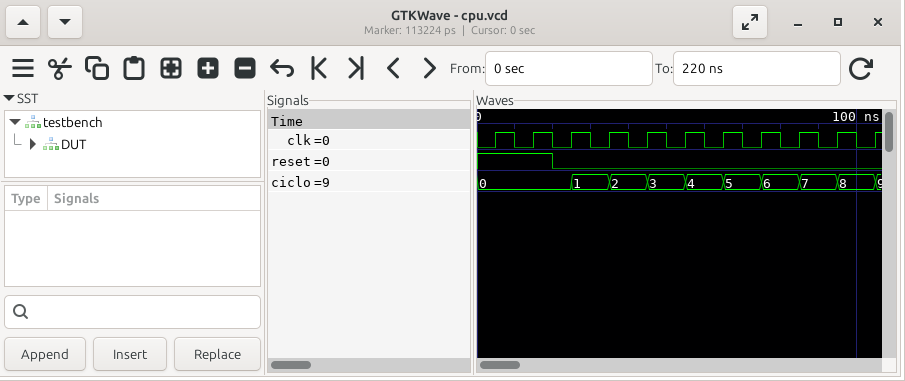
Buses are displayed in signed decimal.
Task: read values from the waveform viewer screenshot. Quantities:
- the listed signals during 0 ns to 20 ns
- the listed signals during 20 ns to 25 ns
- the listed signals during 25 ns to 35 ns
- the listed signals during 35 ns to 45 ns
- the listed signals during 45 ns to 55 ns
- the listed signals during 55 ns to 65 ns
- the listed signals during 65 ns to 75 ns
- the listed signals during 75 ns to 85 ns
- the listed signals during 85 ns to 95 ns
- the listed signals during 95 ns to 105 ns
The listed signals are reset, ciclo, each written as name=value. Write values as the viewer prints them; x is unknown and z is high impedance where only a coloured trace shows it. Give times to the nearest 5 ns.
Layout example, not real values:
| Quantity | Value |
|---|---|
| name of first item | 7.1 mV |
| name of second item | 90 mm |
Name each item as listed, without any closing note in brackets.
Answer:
| Quantity | Value |
|---|---|
| the listed signals during 0 ns to 20 ns | reset=1, ciclo=0 |
| the listed signals during 20 ns to 25 ns | reset=0, ciclo=0 |
| the listed signals during 25 ns to 35 ns | reset=0, ciclo=1 |
| the listed signals during 35 ns to 45 ns | reset=0, ciclo=2 |
| the listed signals during 45 ns to 55 ns | reset=0, ciclo=3 |
| the listed signals during 55 ns to 65 ns | reset=0, ciclo=4 |
| the listed signals during 65 ns to 75 ns | reset=0, ciclo=5 |
| the listed signals during 75 ns to 85 ns | reset=0, ciclo=6 |
| the listed signals during 85 ns to 95 ns | reset=0, ciclo=7 |
| the listed signals during 95 ns to 105 ns | reset=0, ciclo=8 |
